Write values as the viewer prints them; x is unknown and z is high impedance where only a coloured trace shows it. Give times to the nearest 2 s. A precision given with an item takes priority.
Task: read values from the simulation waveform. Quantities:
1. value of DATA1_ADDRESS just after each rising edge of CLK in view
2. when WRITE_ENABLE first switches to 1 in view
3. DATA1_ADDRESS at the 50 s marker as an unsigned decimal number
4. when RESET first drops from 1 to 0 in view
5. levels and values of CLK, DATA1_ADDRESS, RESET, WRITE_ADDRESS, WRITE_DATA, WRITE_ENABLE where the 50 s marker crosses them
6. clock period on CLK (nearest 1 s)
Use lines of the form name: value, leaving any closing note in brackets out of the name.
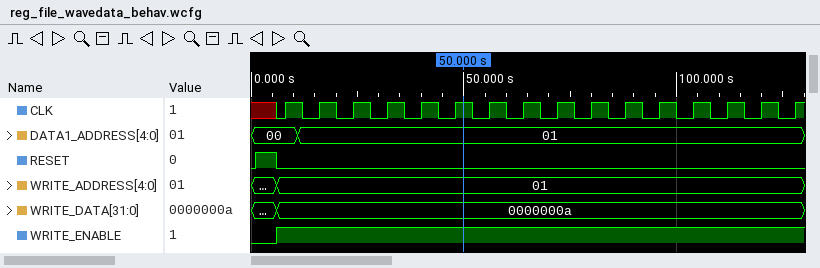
value of DATA1_ADDRESS just after each rising edge of CLK in view: 00, 01, 01, 01, 01, 01, 01, 01, 01, 01, 01, 01, 01, 01, 01, 01
when WRITE_ENABLE first switches to 1 in view: 6 s
DATA1_ADDRESS at the 50 s marker as an unsigned decimal number: 1
when RESET first drops from 1 to 0 in view: 6 s
levels and values of CLK, DATA1_ADDRESS, RESET, WRITE_ADDRESS, WRITE_DATA, WRITE_ENABLE where the 50 s marker crosses them: CLK=1, DATA1_ADDRESS=01, RESET=0, WRITE_ADDRESS=01, WRITE_DATA=0000000a, WRITE_ENABLE=1
clock period on CLK: 8 s
